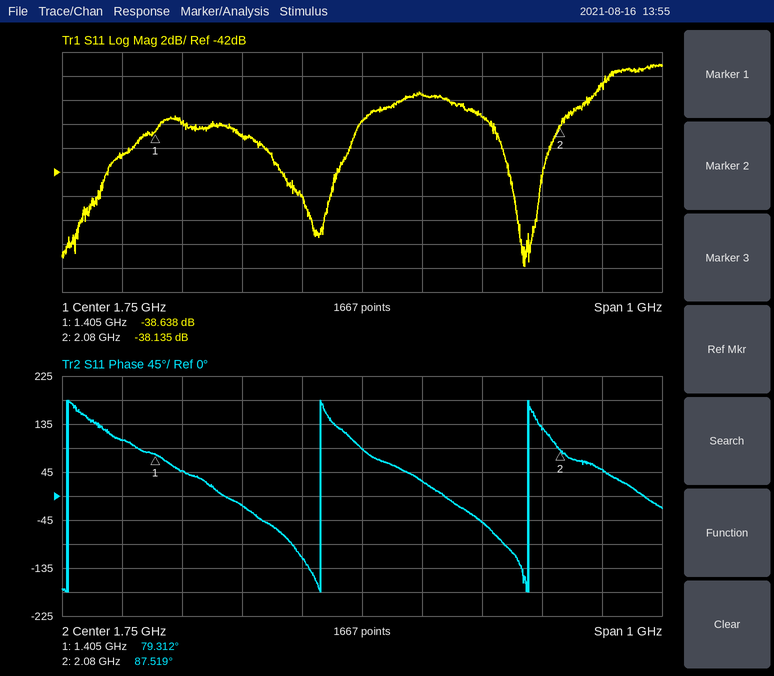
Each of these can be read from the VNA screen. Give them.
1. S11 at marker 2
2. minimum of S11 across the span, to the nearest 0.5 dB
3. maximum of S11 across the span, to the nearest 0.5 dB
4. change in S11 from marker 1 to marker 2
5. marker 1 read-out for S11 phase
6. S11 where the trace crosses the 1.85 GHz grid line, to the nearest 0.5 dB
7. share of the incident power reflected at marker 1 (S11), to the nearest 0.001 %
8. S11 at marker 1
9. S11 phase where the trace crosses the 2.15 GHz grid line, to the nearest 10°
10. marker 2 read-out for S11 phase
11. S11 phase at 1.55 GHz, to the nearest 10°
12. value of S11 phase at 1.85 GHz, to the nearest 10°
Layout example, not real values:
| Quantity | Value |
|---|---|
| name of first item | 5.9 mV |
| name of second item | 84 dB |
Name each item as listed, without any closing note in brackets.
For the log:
| Quantity | Value |
|---|---|
| S11 at marker 2 | -38.135 dB |
| minimum of S11 across the span, to the nearest 0.5 dB | -50.0 dB |
| maximum of S11 across the span, to the nearest 0.5 dB | -33.0 dB |
| change in S11 from marker 1 to marker 2 | 0.503 dB |
| marker 1 read-out for S11 phase | 79.312° |
| S11 where the trace crosses the 1.85 GHz grid line, to the nearest 0.5 dB | -35.5 dB |
| share of the incident power reflected at marker 1 (S11), to the nearest 0.001 % | 0.014 % |
| S11 at marker 1 | -38.638 dB |
| S11 phase where the trace crosses the 2.15 GHz grid line, to the nearest 10° | 50° |
| marker 2 read-out for S11 phase | 87.519° |
| S11 phase at 1.55 GHz, to the nearest 10° | -20° |
| value of S11 phase at 1.85 GHz, to the nearest 10° | 30° |
